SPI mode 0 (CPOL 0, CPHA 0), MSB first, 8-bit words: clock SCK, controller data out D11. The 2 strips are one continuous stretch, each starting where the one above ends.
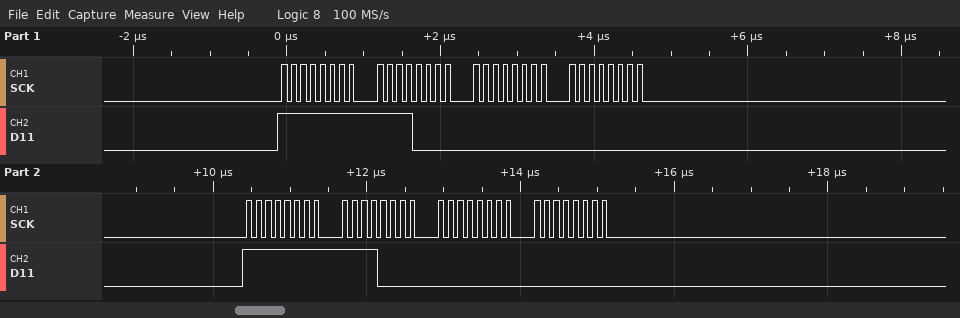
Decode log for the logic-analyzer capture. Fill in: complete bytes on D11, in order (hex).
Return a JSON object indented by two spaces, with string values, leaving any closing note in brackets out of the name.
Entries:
{
  "complete bytes on D11, in order": "FF F0 00 00 FF F0 00 00"
}
